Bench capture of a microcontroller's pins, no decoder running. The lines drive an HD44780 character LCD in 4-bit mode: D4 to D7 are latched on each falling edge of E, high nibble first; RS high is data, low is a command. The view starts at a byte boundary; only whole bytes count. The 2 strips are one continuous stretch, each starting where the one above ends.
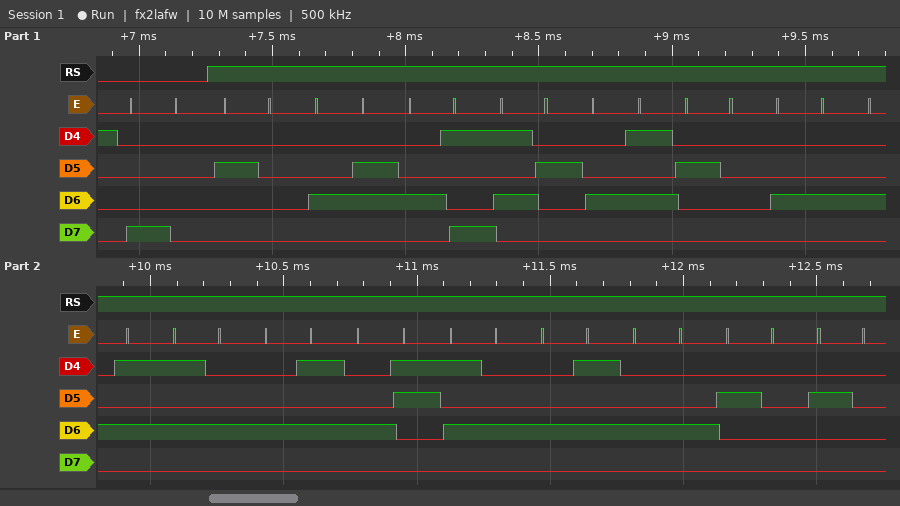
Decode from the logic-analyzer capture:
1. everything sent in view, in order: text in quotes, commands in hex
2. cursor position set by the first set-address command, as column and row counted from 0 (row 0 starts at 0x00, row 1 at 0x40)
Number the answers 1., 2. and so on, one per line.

1. 0x80 " FIRE DETECTED  "
2. column 0, row 0
